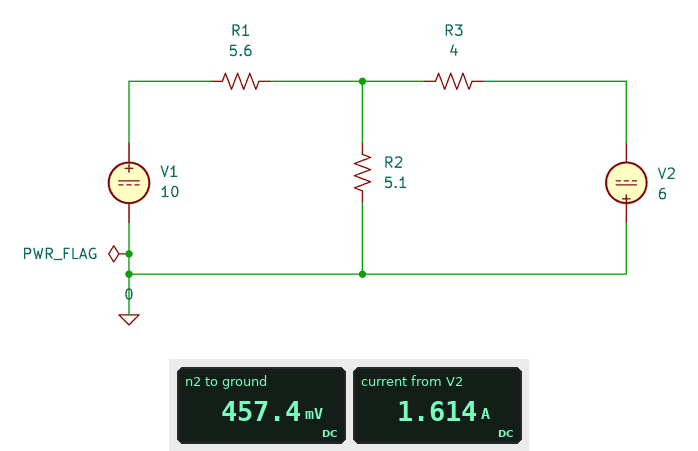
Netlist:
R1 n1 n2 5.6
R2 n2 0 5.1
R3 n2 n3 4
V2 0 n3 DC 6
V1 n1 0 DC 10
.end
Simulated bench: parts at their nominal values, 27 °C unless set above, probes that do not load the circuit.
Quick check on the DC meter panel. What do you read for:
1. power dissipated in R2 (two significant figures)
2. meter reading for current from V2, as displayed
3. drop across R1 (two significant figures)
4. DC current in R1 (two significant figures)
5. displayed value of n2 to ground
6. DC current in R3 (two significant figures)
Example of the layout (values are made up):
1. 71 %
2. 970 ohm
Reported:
1. 41 mW
2. 1.614 A
3. 9.5 V
4. 1.7 A
5. 457.4 mV
6. 1.6 A
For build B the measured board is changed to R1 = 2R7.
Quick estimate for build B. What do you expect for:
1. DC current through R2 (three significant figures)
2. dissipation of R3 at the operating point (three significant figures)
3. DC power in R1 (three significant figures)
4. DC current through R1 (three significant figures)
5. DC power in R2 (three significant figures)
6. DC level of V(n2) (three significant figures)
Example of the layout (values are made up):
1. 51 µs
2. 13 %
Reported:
1. 529 mA
2. 18.9 W
3. 19.7 W
4. 2.70 A
5. 1.43 W
6. 2.70 V
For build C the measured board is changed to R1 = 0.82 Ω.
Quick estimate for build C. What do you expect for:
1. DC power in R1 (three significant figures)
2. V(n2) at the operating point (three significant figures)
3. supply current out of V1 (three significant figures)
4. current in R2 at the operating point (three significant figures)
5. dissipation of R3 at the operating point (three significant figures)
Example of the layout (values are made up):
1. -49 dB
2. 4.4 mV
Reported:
1. 15.6 W
2. 6.42 V
3. 4.36 A
4. 1.26 A
5. 38.6 W
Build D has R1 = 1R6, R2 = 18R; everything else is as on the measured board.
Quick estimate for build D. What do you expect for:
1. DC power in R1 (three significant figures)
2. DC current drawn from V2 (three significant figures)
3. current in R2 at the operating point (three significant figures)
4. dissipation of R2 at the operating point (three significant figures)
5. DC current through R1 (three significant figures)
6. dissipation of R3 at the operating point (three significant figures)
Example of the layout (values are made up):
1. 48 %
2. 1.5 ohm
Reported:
1. 15.0 W
2. 2.78 A
3. 284 mA
4. 1.45 W
5. 3.06 A
6. 30.8 W
